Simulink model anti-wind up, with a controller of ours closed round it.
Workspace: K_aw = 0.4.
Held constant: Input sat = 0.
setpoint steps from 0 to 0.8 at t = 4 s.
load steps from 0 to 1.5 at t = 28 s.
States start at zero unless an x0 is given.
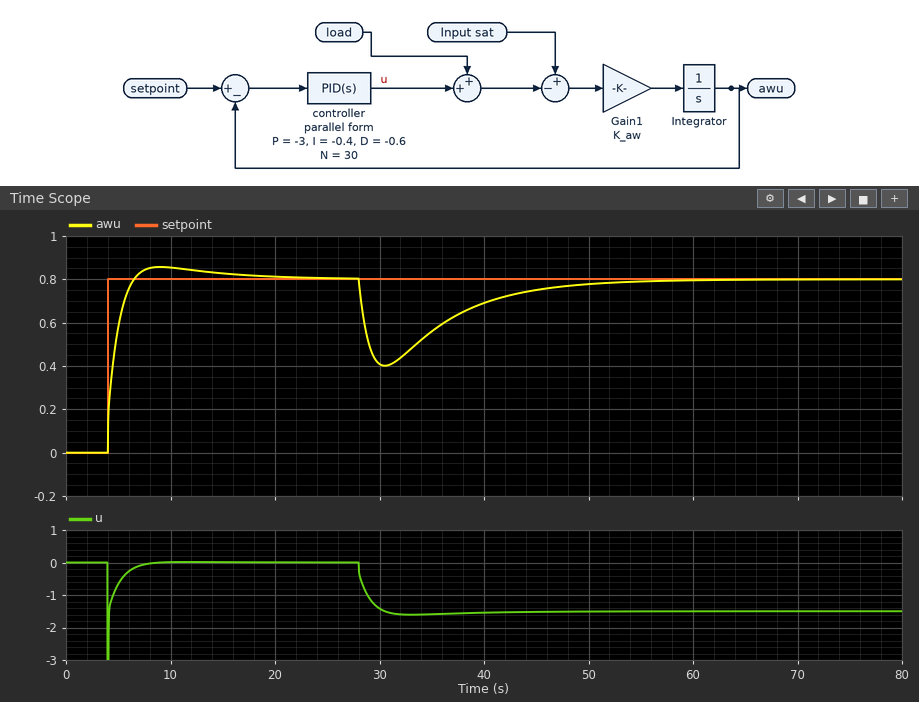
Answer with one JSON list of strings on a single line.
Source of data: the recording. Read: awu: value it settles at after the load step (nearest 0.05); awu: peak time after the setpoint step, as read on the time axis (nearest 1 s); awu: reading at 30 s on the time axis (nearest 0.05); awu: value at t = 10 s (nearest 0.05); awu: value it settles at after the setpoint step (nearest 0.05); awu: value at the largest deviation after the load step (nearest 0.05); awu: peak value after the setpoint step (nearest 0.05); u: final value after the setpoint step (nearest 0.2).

["0.80", "9 s", "0.40", "0.85", "0.80", "0.40", "0.85", "0.0"]
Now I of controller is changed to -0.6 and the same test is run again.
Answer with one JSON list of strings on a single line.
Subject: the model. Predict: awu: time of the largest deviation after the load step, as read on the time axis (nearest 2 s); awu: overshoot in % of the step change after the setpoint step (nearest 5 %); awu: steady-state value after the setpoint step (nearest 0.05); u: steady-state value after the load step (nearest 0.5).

["30 s", "10 %", "0.80", "-1.5"]
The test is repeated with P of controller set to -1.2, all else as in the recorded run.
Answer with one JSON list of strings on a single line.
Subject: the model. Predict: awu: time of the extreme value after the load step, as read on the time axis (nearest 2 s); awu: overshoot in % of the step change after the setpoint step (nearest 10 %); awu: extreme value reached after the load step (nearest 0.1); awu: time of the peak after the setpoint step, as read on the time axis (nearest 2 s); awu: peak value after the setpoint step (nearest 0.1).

["32 s", "20 %", "0.1", "10 s", "1.0"]
